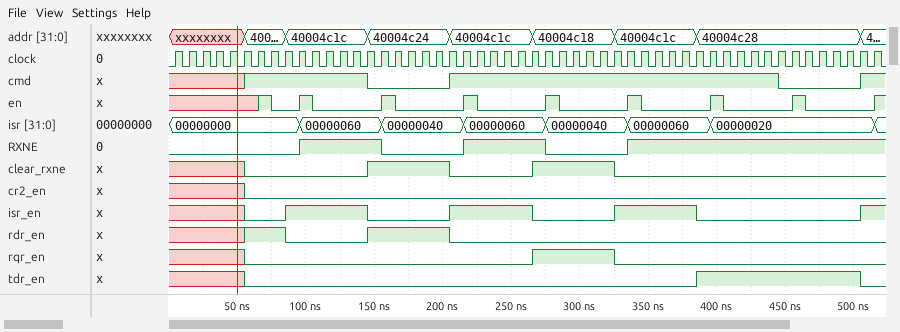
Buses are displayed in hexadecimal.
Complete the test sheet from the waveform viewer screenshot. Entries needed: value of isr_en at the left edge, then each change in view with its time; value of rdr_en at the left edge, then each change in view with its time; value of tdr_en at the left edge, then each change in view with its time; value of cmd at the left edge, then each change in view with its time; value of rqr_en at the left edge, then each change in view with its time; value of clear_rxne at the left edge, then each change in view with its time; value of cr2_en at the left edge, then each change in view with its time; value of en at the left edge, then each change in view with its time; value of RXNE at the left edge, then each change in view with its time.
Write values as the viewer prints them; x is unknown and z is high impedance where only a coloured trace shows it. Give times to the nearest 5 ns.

x, 0 at 55 ns, 1 at 85 ns, 0 at 145 ns, 1 at 205 ns, 0 at 265 ns, 1 at 325 ns, 0 at 385 ns, 1 at 505 ns
x, 1 at 55 ns, 0 at 85 ns, 1 at 145 ns, 0 at 205 ns
x, 0 at 55 ns, 1 at 385 ns, 0 at 505 ns
x, 1 at 55 ns, 0 at 145 ns, 1 at 205 ns, 0 at 445 ns, 1 at 505 ns
x, 0 at 55 ns, 1 at 265 ns, 0 at 325 ns
x, 0 at 55 ns, 1 at 145 ns, 0 at 205 ns, 1 at 265 ns, 0 at 325 ns
x, 0 at 55 ns
x, 1 at 65 ns, 0 at 75 ns, 1 at 95 ns, 0 at 105 ns, 1 at 155 ns, 0 at 165 ns, 1 at 215 ns, 0 at 225 ns, 1 at 275 ns, 0 at 285 ns, 1 at 335 ns, 0 at 345 ns, 1 at 395 ns, 0 at 405 ns, 1 at 455 ns, 0 at 465 ns, 1 at 515 ns
0, 1 at 95 ns, 0 at 155 ns, 1 at 215 ns, 0 at 275 ns, 1 at 335 ns
